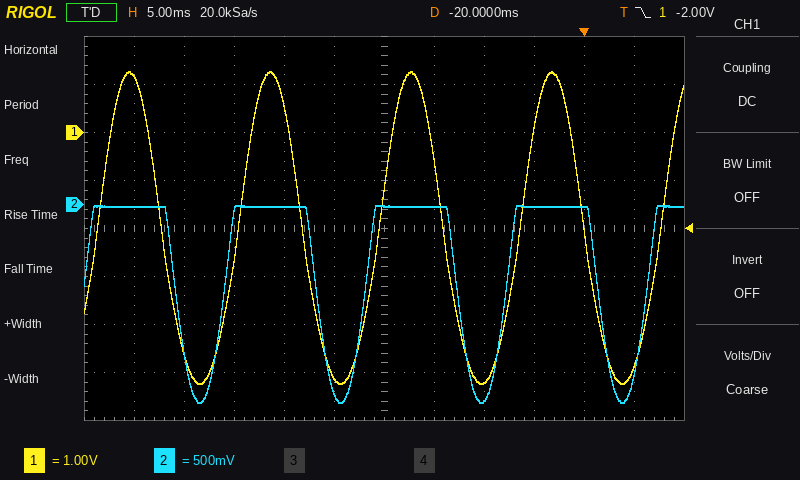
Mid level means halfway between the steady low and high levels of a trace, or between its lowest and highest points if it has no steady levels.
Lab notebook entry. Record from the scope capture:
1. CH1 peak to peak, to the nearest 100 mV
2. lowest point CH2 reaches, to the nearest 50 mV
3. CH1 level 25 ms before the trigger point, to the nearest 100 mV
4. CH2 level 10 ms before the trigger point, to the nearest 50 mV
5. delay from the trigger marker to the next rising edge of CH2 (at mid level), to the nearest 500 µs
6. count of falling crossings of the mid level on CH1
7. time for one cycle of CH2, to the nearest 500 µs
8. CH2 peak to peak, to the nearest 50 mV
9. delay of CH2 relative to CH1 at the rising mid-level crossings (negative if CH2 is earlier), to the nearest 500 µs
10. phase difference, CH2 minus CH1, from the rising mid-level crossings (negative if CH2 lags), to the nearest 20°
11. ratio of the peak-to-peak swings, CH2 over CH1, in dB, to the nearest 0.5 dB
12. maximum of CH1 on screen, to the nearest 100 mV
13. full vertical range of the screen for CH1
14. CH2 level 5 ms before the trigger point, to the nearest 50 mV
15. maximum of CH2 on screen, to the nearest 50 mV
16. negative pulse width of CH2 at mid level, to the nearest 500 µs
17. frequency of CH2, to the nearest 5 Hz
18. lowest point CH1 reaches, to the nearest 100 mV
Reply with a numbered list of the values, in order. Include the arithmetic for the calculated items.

1. 1.3 V − (-5.2 V) = 6.5 V
2. -2.05 V
3. -5.1 V
4. -2.05 V
5. 6.0 ms
6. 4
7. 14.0 ms
8. 0 mV − (-2.05 V) = 2.05 V
9. -1.5 ms
10. −360° × (-1.5 ms) / 14.0 ms ≈ +38.6°, so +40° to the nearest 20°
11. 20 log10(2.05 V / 6.5 V) ≈ -10.0 dB
12. 1.3 V
13. 8 V
14. 0 mV
15. 0 mV
16. 4.5 ms
17. 1 / 14.0 ms ≈ 71.4 Hz, so 70 Hz to the nearest 5 Hz
18. -5.2 V
